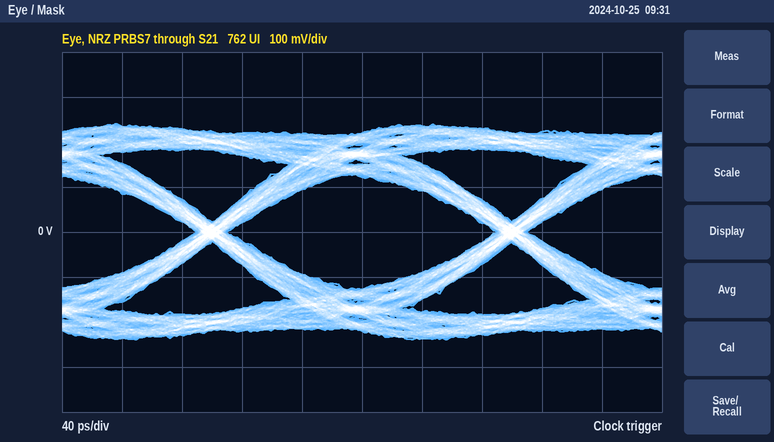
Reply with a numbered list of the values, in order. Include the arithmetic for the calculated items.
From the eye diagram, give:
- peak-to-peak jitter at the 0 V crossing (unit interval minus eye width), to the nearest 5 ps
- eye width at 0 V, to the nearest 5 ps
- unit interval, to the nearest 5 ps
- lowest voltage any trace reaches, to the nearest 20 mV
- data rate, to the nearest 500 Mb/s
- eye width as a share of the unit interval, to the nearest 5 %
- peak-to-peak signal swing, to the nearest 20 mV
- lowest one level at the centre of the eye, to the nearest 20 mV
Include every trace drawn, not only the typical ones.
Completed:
1. 20 ps
2. 180 ps
3. 200 ps
4. -240 mV
5. 5.0 Gb/s
6. 180 ps / 200 ps ≈ 90 %
7. 480 mV
8. 120 mV
